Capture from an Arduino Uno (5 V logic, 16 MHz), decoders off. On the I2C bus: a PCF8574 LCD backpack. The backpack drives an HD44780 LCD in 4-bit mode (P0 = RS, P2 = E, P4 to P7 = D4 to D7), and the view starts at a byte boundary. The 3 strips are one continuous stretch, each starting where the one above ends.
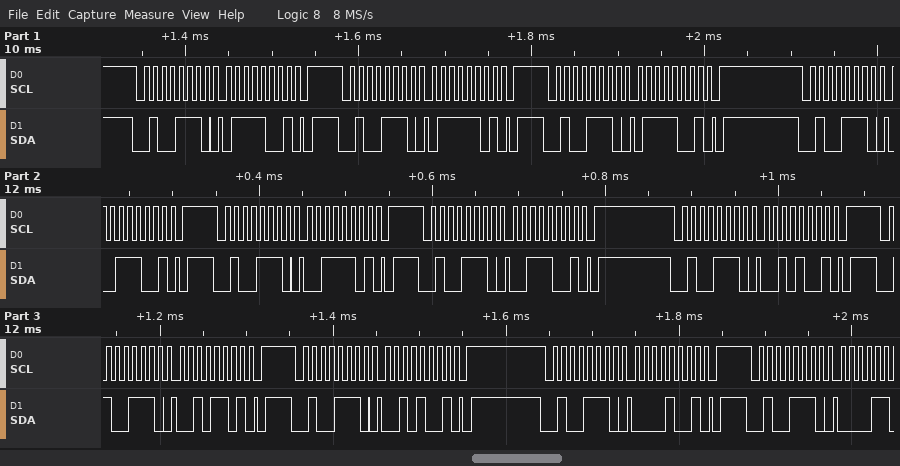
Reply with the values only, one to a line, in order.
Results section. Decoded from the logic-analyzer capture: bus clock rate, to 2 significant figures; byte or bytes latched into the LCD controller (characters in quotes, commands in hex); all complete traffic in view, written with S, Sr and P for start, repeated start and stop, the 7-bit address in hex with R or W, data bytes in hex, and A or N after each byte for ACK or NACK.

100 kHz
's'
S 27W A 79 A P S 27W A 7D A P S 27W A 79 A P S 27W A 39 A P S 27W A 3D A P S 27W A 39 A P S 27W A 29 A P S 27W A 2D A P S 27W A 29 A P S 27W A 09 A P S 27W A
